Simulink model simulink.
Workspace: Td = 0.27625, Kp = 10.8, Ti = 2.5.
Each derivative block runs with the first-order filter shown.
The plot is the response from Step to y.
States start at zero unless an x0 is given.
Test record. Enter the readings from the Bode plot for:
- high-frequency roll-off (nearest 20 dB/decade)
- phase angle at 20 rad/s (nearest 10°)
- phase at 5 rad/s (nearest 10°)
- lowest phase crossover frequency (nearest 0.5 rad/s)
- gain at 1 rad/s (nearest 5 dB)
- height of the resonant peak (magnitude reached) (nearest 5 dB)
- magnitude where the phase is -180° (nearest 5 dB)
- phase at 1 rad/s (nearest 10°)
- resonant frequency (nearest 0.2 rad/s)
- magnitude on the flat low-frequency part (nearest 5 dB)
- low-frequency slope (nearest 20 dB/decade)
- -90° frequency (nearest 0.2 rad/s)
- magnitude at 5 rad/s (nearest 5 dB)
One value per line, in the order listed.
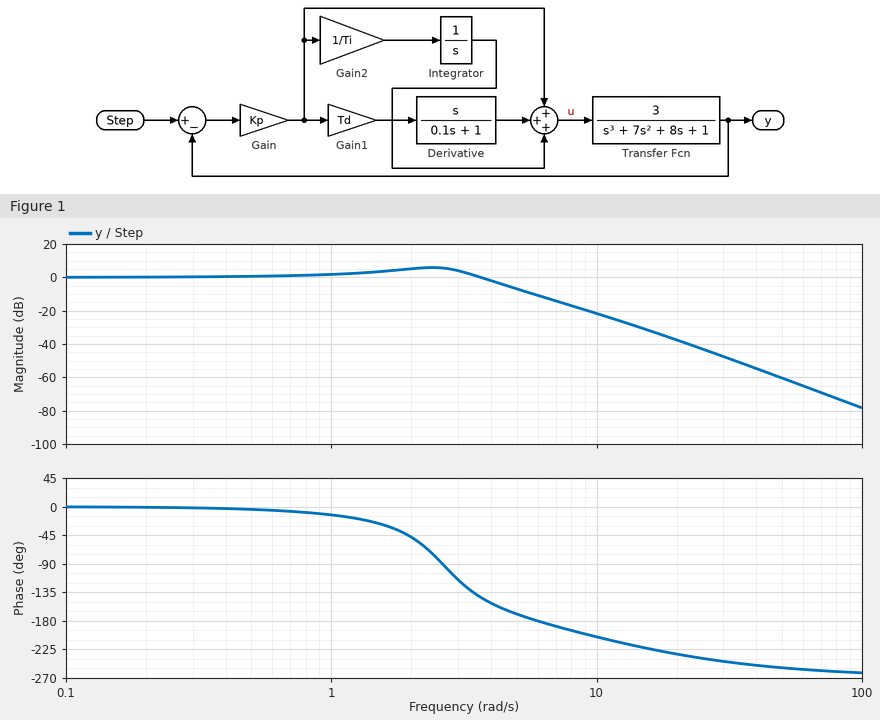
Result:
-60 dB/decade
-230°
-170°
6.0 rad/s
0 dB
5 dB
-10 dB
-10°
2.4 rad/s
0 dB
0 dB/decade
2.6 rad/s
-5 dB
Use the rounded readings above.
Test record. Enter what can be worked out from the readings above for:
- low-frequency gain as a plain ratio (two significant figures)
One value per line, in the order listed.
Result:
1.0
